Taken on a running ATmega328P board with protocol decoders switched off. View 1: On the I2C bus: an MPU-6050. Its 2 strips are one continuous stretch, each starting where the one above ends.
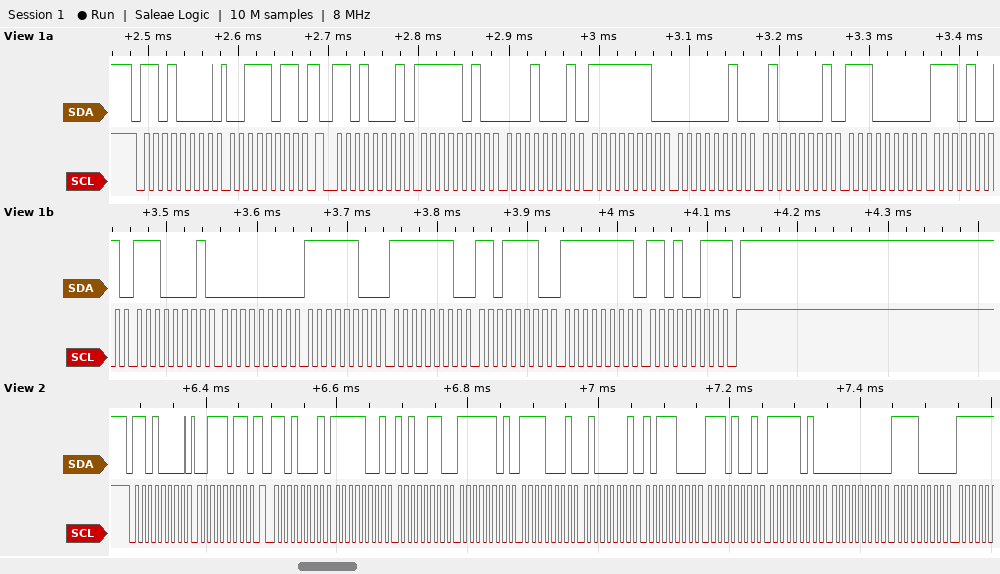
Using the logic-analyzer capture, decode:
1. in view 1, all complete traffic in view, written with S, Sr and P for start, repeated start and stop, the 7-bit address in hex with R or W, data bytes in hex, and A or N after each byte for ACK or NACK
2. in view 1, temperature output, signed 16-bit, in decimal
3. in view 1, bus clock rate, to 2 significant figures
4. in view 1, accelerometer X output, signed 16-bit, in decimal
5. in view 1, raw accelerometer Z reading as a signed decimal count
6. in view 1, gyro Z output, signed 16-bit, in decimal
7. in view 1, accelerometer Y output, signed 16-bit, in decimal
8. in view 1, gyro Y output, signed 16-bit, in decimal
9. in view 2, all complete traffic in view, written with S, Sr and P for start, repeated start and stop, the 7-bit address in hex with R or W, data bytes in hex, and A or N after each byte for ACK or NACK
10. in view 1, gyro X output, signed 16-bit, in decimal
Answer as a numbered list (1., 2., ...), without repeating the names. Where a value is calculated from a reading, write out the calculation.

1. S 68W A 3B A Sr 68R A FA A 11 A FE A 02 A 41 A E0 A E9 A E1 A 00 A FC A FE A DE A FF A D3 N P
2. 0xE9E1 = -5663
3. 100 kHz
4. 0xFA11 = -1519
5. 0x41E0 = 16864
6. 0xFFD3 = -45
7. 0xFE02 = -510
8. 0xFEDE = -290
9. S 68W A 3B A Sr 68R A F9 A A6 A FD A F1 A 41 A B8 A E9 A FA A 00 A F0 A
10. 0x00FC = 252
